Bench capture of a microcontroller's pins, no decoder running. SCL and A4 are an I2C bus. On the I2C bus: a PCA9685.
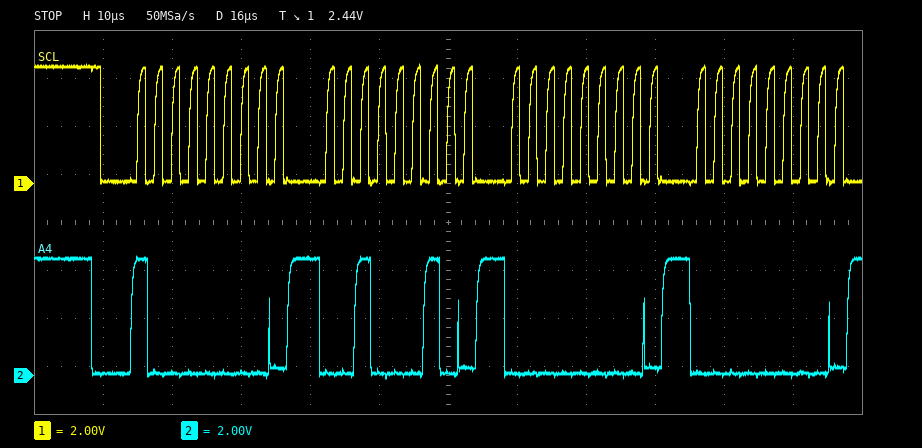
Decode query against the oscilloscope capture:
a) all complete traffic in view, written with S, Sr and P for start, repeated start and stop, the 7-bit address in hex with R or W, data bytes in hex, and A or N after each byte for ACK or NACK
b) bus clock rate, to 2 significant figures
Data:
S 40W A 22 A 00 A 00 A
400 kHz
